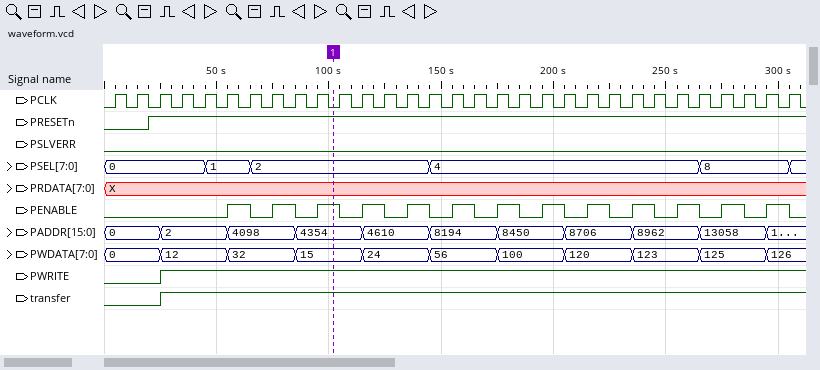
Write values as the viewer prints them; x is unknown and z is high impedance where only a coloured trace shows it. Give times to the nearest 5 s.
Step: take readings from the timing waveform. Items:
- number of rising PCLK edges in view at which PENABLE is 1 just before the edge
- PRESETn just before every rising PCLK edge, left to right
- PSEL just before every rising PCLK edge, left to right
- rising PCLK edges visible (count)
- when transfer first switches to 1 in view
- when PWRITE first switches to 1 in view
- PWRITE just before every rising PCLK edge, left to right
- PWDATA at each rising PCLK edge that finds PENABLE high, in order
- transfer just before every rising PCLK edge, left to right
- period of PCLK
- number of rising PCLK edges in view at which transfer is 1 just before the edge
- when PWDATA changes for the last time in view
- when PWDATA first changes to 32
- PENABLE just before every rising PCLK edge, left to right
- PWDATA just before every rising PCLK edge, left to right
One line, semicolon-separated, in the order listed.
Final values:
13; 0 0 1 1 1 1 1 1 1 1 1 1 1 1 1 1 1 1 1 1 1 1 1 1 1 1 1 1 1 1 1; 0, 0, 0, 0, 0, 1, 1, 2, 2, 2, 2, 2, 2, 2, 2, 4, 4, 4, 4, 4, 4, 4, 4, 4, 4, 4, 4, 8, 8, 8, 8; 31; 25 s; 25 s; 0 0 0 1 1 1 1 1 1 1 1 1 1 1 1 1 1 1 1 1 1 1 1 1 1 1 1 1 1 1 1; 32, 32, 15, 24, 24, 56, 100, 100, 120, 123, 123, 125, 126; 0 0 0 1 1 1 1 1 1 1 1 1 1 1 1 1 1 1 1 1 1 1 1 1 1 1 1 1 1 1 1; 10 s; 28; 295 s; 55 s; 0 0 0 0 0 0 1 0 1 0 1 0 1 0 1 0 1 0 1 0 1 0 1 0 1 0 1 0 1 0 1; 0, 0, 0, 12, 12, 12, 32, 32, 32, 15, 15, 15, 24, 24, 24, 56, 56, 56, 100, 100, 100, 120, 120, 120, 123, 123, 123, 125, 125, 125, 126
